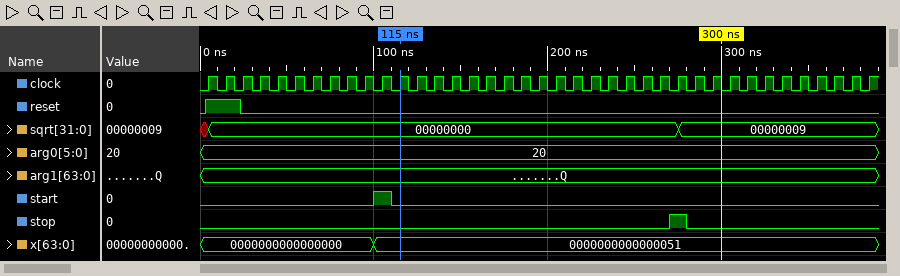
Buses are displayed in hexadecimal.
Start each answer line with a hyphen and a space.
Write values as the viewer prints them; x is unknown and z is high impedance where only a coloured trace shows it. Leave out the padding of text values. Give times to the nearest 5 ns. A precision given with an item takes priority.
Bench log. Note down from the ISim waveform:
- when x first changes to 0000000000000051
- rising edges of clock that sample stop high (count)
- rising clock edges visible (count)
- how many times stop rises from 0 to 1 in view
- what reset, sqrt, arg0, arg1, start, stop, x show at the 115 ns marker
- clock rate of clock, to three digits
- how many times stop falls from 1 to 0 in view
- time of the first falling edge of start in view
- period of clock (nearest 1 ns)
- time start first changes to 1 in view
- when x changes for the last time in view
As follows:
- 100 ns
- 1
- 39
- 1
- reset=0, sqrt=00000000, arg0=20, arg1=Q, start=0, stop=0, x=0000000000000051
- 100 MHz
- 1
- 110 ns
- 10 ns
- 100 ns
- 100 ns
